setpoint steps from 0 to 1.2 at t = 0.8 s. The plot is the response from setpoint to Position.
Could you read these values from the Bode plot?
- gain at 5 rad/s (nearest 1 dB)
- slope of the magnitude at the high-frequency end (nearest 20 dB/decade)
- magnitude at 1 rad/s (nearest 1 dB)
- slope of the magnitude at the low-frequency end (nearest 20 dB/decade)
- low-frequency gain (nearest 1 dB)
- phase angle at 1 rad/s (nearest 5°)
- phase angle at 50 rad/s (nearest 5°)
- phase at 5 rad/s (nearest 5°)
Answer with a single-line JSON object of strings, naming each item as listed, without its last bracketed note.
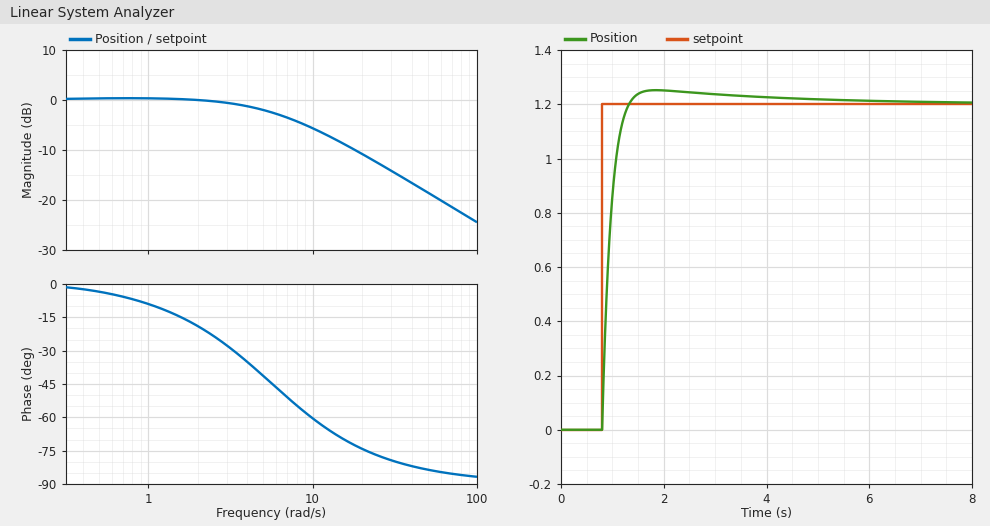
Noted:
{"gain at 5 rad/s": "-2 dB", "slope of the magnitude at the high-frequency end": "-20 dB/decade", "magnitude at 1 rad/s": "0 dB", "slope of the magnitude at the low-frequency end": "0 dB/decade", "low-frequency gain": "0 dB", "phase angle at 1 rad/s": "-10°", "phase angle at 50 rad/s": "-85°", "phase at 5 rad/s": "-40°"}
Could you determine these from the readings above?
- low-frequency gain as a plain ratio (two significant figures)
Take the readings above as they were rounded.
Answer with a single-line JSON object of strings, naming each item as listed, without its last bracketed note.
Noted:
{"low-frequency gain as a plain ratio": "1.0"}
